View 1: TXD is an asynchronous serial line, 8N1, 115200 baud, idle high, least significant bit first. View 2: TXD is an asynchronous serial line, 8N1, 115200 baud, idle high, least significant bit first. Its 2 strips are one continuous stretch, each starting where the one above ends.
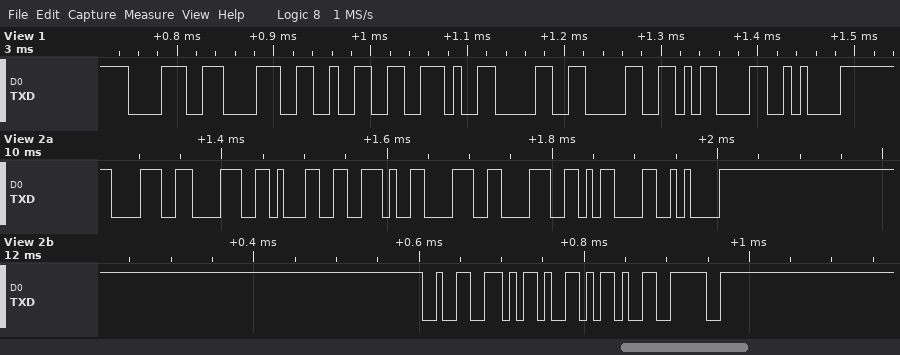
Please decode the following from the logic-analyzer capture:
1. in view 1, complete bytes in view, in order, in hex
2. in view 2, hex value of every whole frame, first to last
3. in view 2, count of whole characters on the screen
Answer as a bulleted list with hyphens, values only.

- 38 38 32 2E 30 30 0D 0A
- 0x38 0x38 0x31 0x2E 0x38 0x38 0x0D 0x0A 0x32 0x2D 0x2D 0x3E
- 12
